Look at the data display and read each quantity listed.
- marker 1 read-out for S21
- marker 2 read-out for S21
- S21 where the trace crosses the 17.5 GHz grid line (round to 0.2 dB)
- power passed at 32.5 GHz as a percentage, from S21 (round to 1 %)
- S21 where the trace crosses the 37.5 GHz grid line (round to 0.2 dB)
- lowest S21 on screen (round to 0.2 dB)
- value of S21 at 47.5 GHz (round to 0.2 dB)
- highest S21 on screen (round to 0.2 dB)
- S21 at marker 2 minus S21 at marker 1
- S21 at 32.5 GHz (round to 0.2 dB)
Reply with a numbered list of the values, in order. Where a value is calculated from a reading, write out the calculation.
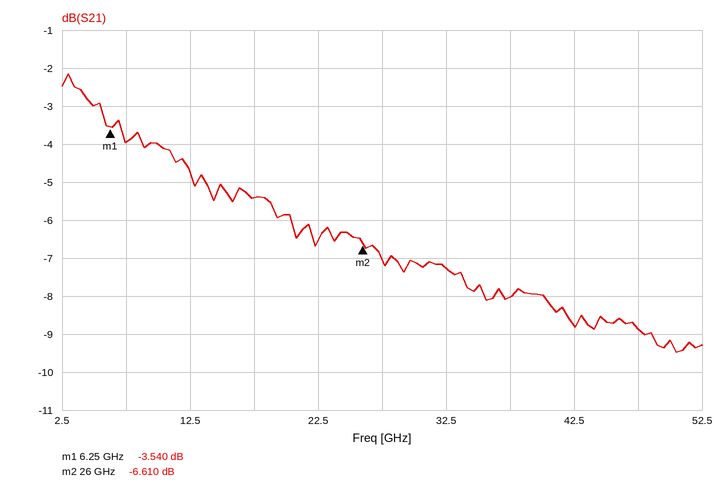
1. -3.540 dB
2. -6.610 dB
3. -5.4 dB
4. 10^(-7.2/10) ≈ 19 %
5. -8.0 dB
6. -9.4 dB
7. -8.8 dB
8. -2.2 dB
9. -6.61 − (-3.54) = -3.070 dB
10. -7.2 dB
